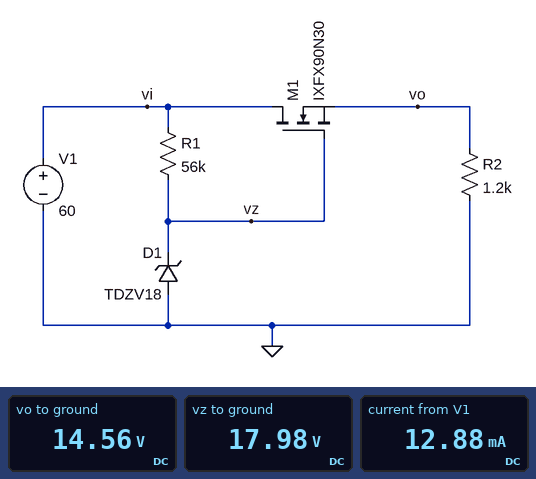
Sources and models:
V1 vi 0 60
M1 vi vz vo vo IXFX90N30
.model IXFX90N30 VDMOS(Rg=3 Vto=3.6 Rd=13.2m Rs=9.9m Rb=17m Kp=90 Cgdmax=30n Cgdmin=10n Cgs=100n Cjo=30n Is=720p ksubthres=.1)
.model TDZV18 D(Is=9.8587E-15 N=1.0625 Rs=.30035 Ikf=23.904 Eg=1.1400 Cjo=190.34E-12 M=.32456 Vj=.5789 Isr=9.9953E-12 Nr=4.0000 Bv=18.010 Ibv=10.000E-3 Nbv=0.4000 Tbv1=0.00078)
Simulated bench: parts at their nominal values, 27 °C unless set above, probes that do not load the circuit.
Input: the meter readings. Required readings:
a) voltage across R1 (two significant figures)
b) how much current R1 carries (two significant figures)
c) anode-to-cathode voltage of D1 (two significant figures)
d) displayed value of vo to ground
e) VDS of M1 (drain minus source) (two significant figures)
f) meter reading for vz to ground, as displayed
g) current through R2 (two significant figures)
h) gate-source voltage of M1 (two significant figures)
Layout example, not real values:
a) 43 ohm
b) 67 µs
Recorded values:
a) 42 V
b) 750 µA
c) -18 V
d) 14.56 V
e) 45 V
f) 17.98 V
g) 12 mA
h) 3.4 V
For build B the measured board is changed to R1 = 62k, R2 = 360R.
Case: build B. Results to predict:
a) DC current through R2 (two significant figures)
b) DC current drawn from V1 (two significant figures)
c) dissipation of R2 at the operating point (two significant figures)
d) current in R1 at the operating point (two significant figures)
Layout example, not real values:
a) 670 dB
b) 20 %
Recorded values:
a) 40 mA
b) 41 mA
c) 580 mW
d) 680 µA
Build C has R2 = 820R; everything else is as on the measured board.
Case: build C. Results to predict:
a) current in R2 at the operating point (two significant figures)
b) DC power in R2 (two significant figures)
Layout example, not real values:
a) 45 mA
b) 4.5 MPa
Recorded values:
a) 18 mA
b) 260 mW
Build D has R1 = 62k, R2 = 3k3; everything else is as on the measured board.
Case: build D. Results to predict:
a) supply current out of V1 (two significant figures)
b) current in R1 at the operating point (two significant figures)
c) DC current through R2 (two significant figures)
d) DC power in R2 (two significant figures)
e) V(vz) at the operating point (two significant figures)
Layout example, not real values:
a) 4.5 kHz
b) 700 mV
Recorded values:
a) 5.1 mA
b) 680 µA
c) 4.4 mA
d) 65 mW
e) 18 V
